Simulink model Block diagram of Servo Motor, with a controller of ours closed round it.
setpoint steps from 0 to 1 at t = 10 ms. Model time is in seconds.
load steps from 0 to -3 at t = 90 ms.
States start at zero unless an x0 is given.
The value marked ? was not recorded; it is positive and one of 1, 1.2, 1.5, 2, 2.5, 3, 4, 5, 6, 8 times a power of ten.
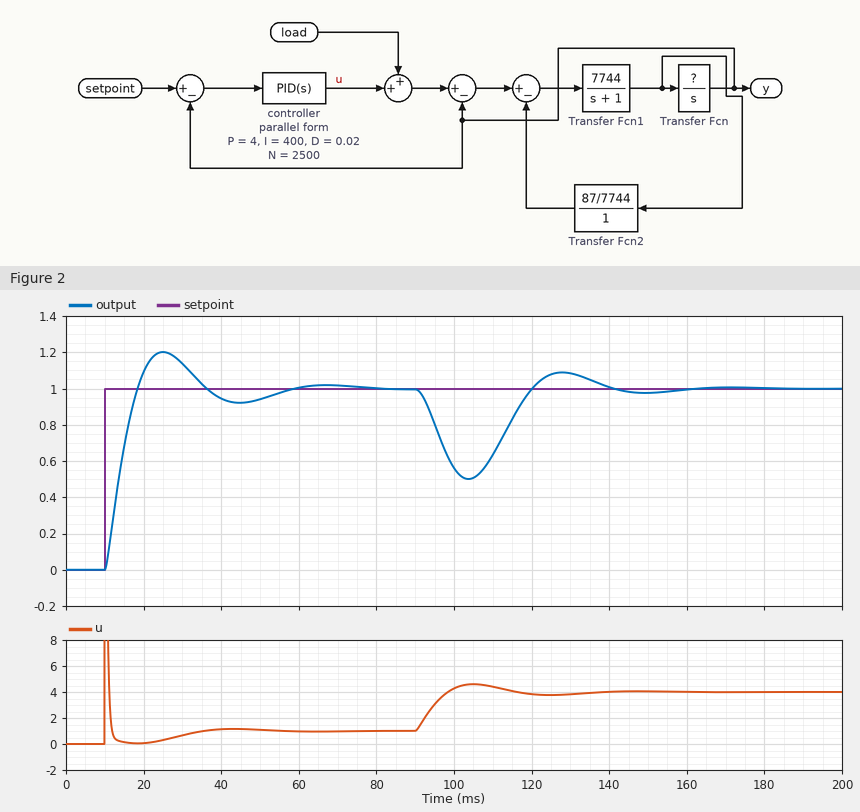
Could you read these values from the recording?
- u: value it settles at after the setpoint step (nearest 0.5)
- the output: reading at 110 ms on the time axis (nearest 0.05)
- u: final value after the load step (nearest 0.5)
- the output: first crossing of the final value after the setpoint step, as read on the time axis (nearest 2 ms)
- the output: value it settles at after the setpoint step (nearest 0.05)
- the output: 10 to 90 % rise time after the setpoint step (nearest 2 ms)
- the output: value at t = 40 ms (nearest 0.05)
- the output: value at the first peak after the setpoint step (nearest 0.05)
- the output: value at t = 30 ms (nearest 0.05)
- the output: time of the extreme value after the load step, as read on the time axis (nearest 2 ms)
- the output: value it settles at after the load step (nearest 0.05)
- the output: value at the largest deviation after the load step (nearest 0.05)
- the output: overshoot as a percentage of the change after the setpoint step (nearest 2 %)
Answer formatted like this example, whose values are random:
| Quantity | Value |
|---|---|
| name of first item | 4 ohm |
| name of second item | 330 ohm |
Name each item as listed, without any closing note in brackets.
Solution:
| Quantity | Value |
|---|---|
| u: value it settles at after the setpoint step | 1.0 |
| the output: reading at 110 ms on the time axis | 0.65 |
| u: final value after the load step | 4.0 |
| the output: first crossing of the final value after the setpoint step, as read on the time axis | 18 ms |
| the output: value it settles at after the setpoint step | 1.00 |
| the output: 10 to 90 % rise time after the setpoint step | 6 ms |
| the output: value at t = 40 ms | 0.95 |
| the output: value at the first peak after the setpoint step | 1.20 |
| the output: value at t = 30 ms | 1.15 |
| the output: time of the extreme value after the load step, as read on the time axis | 104 ms |
| the output: value it settles at after the load step | 1.00 |
| the output: value at the largest deviation after the load step | 0.50 |
| the output: overshoot as a percentage of the change after the setpoint step | 20 % |
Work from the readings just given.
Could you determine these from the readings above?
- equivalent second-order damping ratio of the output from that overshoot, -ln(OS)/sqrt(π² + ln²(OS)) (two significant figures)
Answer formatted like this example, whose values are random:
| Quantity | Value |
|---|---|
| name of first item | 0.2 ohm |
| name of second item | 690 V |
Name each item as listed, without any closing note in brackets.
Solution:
| Quantity | Value |
|---|---|
| equivalent second-order damping ratio of the output from that overshoot, -ln(OS)/sqrt(π² + ln²(OS)) | 0.46 |
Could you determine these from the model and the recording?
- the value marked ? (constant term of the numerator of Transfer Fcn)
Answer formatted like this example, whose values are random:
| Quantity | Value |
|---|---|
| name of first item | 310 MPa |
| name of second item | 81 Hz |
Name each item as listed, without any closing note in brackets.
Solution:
| Quantity | Value |
|---|---|
| the value marked ? | 1 |
